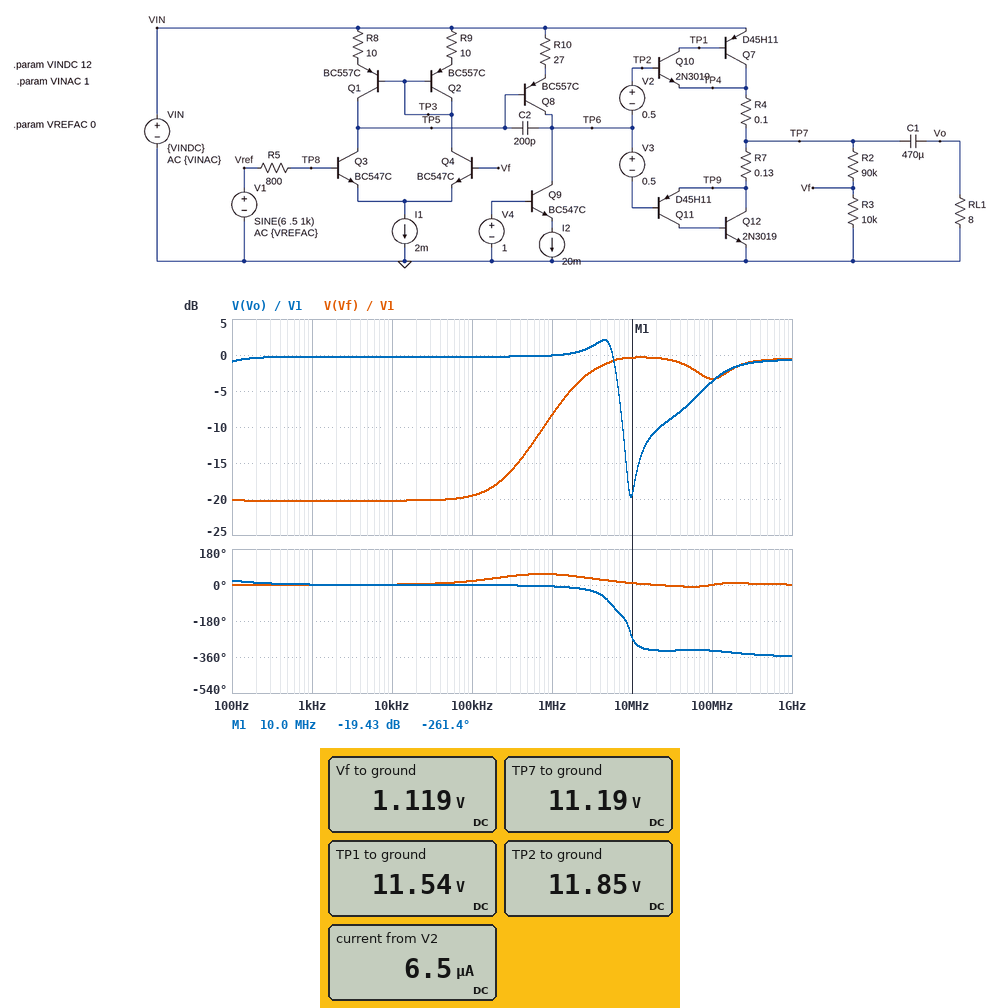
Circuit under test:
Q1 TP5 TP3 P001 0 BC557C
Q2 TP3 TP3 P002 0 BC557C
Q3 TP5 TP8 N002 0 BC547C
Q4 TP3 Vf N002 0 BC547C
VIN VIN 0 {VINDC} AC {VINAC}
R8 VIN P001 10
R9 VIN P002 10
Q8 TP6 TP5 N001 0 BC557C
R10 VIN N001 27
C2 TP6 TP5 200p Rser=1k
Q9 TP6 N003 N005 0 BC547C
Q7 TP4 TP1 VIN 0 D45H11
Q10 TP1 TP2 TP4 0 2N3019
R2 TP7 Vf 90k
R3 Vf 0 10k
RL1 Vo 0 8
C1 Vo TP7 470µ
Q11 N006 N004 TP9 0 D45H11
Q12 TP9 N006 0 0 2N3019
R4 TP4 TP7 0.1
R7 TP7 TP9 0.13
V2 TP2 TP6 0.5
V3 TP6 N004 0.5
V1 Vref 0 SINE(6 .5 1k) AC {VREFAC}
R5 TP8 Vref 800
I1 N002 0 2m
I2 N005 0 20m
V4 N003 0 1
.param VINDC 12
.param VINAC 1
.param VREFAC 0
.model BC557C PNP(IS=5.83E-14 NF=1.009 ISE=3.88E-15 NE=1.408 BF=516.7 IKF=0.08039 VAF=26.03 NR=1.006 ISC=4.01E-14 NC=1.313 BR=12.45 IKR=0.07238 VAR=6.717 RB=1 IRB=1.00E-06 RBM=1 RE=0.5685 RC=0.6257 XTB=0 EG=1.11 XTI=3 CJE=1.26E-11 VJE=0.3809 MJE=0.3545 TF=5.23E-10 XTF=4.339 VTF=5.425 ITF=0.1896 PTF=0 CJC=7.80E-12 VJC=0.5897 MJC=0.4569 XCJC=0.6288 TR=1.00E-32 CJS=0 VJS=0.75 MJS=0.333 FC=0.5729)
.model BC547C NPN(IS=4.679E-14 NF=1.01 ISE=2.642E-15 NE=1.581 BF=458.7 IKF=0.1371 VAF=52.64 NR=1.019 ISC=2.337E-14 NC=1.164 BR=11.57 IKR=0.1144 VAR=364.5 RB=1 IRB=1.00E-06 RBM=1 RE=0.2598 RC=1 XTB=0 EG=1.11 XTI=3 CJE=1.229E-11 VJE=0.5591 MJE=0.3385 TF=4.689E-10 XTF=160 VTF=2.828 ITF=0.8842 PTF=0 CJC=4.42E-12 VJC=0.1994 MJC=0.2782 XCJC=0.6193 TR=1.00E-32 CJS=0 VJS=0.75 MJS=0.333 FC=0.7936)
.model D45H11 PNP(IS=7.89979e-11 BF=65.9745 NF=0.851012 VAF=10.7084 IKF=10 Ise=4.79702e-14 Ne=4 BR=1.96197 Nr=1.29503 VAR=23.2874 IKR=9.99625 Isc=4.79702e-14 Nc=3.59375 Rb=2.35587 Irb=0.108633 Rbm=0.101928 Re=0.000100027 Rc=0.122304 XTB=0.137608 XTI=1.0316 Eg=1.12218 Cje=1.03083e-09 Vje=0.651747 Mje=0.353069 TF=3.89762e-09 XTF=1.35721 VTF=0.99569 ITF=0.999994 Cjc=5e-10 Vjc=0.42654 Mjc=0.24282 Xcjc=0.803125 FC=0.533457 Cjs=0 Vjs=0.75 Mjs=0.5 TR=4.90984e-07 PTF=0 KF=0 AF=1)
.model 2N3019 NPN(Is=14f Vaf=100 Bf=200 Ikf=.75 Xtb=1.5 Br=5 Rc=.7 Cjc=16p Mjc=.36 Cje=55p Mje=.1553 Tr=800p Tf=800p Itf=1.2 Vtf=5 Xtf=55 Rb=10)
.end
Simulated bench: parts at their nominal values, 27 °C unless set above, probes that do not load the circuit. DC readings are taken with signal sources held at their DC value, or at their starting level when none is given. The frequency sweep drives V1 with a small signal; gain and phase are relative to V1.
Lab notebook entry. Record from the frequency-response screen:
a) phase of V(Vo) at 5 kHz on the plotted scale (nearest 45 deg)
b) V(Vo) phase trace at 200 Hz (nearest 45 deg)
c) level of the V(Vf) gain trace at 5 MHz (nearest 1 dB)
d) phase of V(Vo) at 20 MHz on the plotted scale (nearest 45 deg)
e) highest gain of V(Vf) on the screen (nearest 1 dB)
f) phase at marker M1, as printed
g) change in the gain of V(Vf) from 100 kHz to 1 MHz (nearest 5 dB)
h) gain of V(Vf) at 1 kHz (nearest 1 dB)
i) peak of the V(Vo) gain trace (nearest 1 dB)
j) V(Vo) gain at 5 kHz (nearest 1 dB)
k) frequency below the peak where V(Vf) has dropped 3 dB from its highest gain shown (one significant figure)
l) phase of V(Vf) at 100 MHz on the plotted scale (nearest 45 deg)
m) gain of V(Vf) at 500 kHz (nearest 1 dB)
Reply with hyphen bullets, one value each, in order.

- 0 deg
- 0 deg
- -1 dB
- -315 deg
- 0 dB
- -261.4 deg
- 10 dB
- -20 dB
- 2 dB
- 0 dB
- 2 MHz
- 0 deg
- -13 dB
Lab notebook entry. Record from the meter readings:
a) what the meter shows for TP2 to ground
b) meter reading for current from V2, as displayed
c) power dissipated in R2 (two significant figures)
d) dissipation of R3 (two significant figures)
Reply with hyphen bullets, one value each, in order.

- 11.85 V
- 6.5 µA
- 1.1 mW
- 130 µW
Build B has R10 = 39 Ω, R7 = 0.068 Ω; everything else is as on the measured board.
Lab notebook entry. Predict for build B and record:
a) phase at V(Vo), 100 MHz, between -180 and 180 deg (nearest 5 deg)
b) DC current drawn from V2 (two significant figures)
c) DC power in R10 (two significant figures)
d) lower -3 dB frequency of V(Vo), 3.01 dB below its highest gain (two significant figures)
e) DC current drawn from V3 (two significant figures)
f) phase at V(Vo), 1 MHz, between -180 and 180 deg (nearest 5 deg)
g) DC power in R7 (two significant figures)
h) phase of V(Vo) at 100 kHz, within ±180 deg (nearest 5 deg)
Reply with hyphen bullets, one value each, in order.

- 35 deg
- 6.9 µA
- 19 mW
- 93 Hz
- 3.8 µA
- -10 deg
- 600 µW
- 0 deg
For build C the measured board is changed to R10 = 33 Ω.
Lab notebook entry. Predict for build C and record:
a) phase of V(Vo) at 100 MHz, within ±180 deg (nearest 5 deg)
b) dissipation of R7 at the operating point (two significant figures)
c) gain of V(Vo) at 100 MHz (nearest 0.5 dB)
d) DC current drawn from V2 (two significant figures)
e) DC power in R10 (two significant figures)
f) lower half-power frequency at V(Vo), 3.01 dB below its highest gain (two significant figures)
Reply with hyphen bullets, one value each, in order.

- 35 deg
- 980 µW
- -4.0 dB
- 6.4 µA
- 16 mW
- 100 Hz
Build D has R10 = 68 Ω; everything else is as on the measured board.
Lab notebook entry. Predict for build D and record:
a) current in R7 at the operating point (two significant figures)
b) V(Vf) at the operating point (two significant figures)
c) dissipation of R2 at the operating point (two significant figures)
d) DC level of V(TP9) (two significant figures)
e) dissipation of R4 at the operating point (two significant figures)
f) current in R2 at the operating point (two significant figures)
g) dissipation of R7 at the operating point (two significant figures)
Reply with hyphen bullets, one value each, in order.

- 88 mA
- 1.0 V
- 950 µW
- 10 V
- 770 µW
- 100 µA
- 1.0 mW
